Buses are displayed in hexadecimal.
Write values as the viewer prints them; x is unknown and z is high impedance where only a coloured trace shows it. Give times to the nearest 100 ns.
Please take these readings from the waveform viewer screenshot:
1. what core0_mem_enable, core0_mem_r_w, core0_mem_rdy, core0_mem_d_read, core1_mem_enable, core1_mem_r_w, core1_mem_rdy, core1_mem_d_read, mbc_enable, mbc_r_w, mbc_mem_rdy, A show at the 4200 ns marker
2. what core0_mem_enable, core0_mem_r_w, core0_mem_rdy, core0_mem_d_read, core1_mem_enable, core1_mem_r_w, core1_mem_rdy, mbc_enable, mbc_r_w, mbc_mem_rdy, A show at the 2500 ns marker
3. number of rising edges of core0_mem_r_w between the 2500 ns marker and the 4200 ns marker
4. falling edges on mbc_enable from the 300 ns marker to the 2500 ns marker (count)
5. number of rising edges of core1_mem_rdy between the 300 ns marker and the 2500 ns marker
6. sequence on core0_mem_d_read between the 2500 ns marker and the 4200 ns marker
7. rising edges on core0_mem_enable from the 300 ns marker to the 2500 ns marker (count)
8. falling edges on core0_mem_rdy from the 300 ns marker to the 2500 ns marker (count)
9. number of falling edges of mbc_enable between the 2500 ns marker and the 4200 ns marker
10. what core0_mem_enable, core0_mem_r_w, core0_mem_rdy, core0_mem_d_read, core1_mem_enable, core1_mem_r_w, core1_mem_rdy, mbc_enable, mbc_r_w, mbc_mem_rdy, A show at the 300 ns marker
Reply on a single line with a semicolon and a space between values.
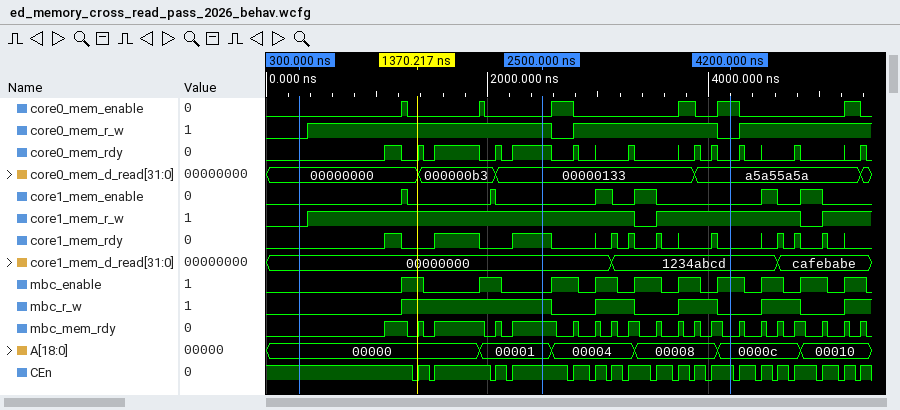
core0_mem_enable=1, core0_mem_r_w=0, core0_mem_rdy=0, core0_mem_d_read=a5a55a5a, core1_mem_enable=0, core1_mem_r_w=1, core1_mem_rdy=0, core1_mem_d_read=1234abcd, mbc_enable=1, mbc_r_w=0, mbc_mem_rdy=0, A=0000c; core0_mem_enable=0, core0_mem_r_w=1, core0_mem_rdy=1, core0_mem_d_read=00000133, core1_mem_enable=0, core1_mem_r_w=1, core1_mem_rdy=1, mbc_enable=0, mbc_r_w=1, mbc_mem_rdy=1, A=00001; 1; 2; 3; 00000133, a5a55a5a; 2; 4; 4; core0_mem_enable=0, core0_mem_r_w=0, core0_mem_rdy=0, core0_mem_d_read=00000000, core1_mem_enable=0, core1_mem_r_w=0, core1_mem_rdy=0, mbc_enable=0, mbc_r_w=0, mbc_mem_rdy=0, A=00000
